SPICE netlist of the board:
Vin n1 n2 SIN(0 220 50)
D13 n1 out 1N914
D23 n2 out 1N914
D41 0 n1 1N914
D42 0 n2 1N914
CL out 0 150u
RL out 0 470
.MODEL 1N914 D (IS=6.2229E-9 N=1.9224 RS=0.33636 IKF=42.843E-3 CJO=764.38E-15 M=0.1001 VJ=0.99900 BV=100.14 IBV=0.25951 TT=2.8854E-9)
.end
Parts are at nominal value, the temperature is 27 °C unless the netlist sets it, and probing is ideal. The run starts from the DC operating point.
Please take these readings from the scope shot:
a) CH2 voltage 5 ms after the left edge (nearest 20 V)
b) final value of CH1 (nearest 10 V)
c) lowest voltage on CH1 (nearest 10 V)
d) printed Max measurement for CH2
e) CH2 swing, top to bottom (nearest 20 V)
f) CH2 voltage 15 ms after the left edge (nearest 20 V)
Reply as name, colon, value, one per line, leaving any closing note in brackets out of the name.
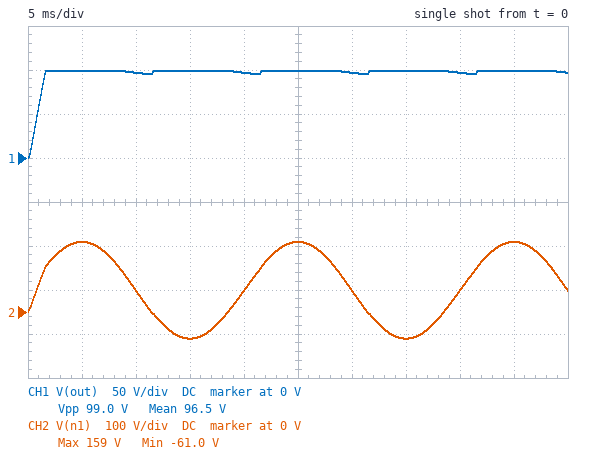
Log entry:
CH2 voltage 5 ms after the left edge: 160 V
final value of CH1: 100 V
lowest voltage on CH1: 0 V
printed Max measurement for CH2: 159 V
CH2 swing, top to bottom: 220 V
CH2 voltage 15 ms after the left edge: -60 V
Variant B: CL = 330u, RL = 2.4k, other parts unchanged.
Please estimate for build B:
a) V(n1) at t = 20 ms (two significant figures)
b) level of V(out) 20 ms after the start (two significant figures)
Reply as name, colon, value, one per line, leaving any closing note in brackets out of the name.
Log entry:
V(n1) at t = 20 ms: 49 V
level of V(out) 20 ms after the start: 99 V
